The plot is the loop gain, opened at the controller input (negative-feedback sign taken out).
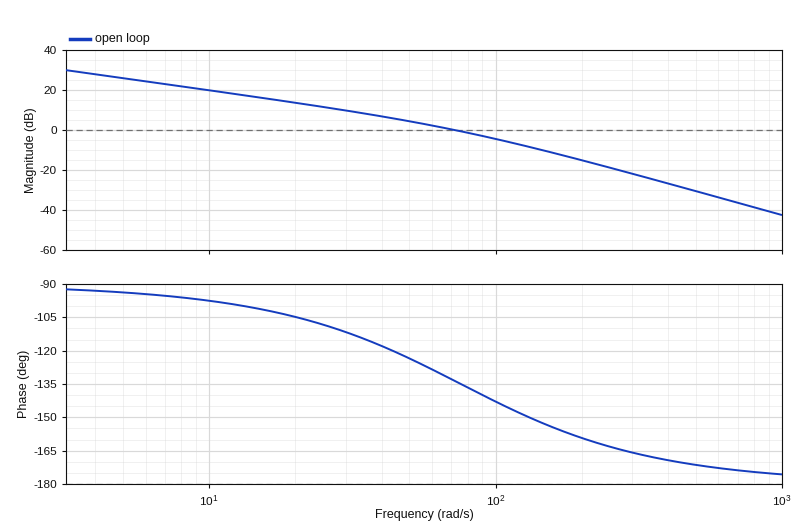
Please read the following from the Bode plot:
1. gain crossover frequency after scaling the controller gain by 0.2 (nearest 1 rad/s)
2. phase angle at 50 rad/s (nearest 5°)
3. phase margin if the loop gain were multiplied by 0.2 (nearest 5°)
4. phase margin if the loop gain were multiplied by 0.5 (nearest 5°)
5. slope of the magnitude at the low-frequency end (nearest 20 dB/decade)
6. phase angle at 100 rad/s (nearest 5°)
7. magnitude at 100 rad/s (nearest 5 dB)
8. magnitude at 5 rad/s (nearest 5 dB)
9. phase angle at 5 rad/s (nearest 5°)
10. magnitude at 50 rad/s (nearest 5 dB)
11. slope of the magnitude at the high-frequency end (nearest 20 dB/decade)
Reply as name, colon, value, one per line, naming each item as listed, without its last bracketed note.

gain crossover frequency after scaling the controller gain by 0.2: 19 rad/s
phase angle at 50 rad/s: -125°
phase margin if the loop gain were multiplied by 0.2: 75°
phase margin if the loop gain were multiplied by 0.5: 60°
slope of the magnitude at the low-frequency end: -20 dB/decade
phase angle at 100 rad/s: -145°
magnitude at 100 rad/s: -5 dB
magnitude at 5 rad/s: 25 dB
phase angle at 5 rad/s: -95°
magnitude at 50 rad/s: 5 dB
slope of the magnitude at the high-frequency end: -40 dB/decade
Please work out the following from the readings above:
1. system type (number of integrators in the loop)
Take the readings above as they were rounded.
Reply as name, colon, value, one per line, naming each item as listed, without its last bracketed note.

system type: 1
